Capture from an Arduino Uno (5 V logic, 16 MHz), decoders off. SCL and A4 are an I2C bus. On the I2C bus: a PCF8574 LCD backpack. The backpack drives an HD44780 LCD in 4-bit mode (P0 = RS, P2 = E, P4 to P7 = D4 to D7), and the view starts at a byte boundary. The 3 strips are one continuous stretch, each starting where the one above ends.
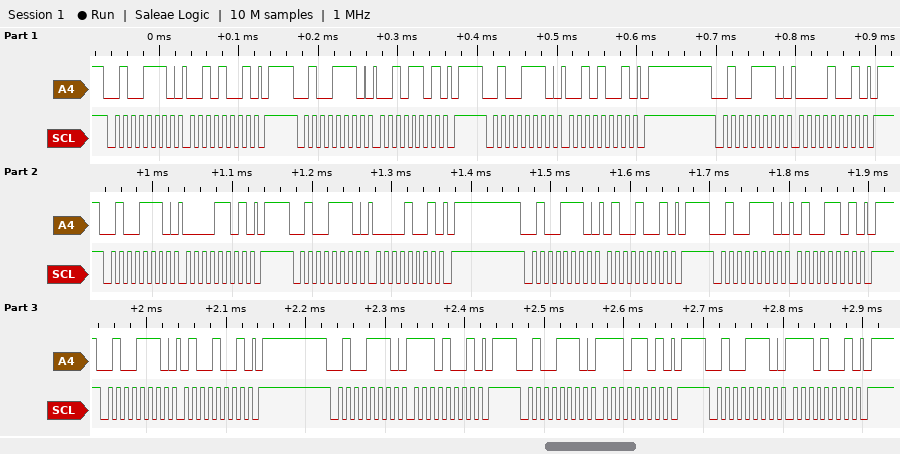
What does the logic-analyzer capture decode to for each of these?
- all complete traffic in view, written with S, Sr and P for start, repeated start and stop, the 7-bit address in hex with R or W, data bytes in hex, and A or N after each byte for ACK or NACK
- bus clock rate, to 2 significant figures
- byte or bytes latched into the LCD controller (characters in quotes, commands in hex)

S 27W A 29 A P S 27W A 2D A P S 27W A 29 A P S 27W A 09 A P S 27W A 0D A P S 27W A 09 A P S 27W A 49 A P S 27W A 4D A P S 27W A 49 A P S 27W A E9 A P S 27W A ED A P S 27W A E9 A P
100 kHz
' ' 'N'
